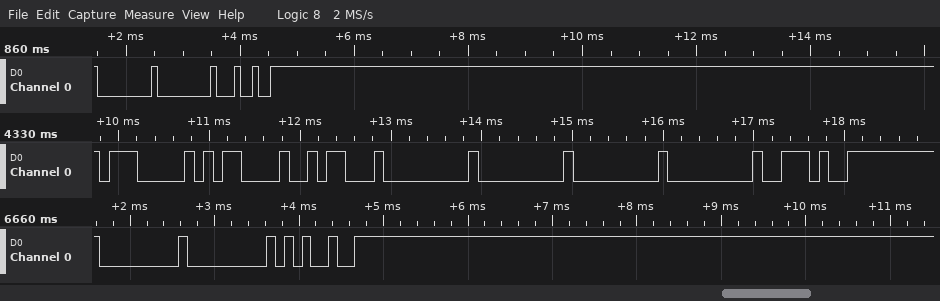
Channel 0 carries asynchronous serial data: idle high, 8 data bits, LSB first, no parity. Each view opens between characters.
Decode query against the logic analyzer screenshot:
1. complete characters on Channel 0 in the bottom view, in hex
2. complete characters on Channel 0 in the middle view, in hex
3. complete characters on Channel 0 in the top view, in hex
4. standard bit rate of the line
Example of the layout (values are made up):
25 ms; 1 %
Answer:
00, 00, 25; 07, 0D, 1A, 00, 00, 00, 00, 2E; 00, 00, 24; 9600 baud
